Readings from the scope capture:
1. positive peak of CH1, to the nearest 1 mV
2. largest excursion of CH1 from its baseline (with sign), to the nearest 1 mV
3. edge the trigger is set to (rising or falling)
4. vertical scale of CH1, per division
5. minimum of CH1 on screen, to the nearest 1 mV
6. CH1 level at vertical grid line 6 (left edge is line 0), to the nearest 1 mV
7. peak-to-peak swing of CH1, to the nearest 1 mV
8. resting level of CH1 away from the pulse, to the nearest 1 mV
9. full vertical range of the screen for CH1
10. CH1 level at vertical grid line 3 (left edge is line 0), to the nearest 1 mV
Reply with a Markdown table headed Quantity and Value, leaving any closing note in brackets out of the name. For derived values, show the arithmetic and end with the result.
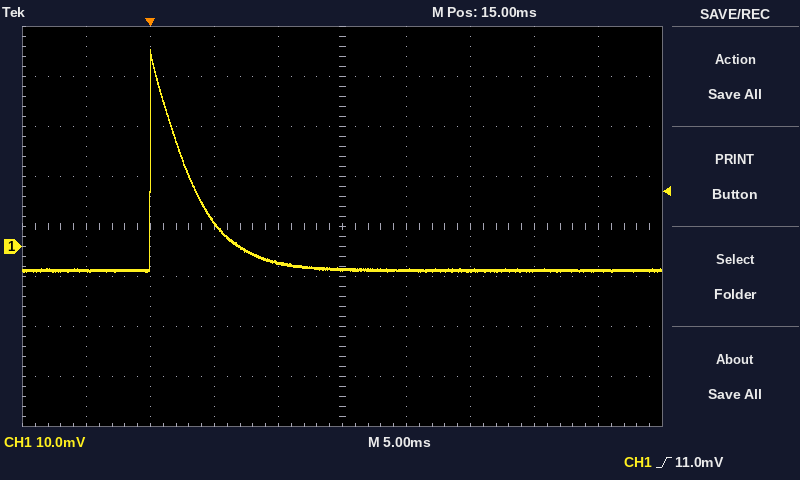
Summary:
| Quantity | Value |
|---|---|
| positive peak of CH1, to the nearest 1 mV | 39 mV |
| largest excursion of CH1 from its baseline (with sign), to the nearest 1 mV | 39 mV − (-5 mV) = +44 mV |
| edge the trigger is set to | rising |
| vertical scale of CH1, per division | 10 mV |
| minimum of CH1 on screen, to the nearest 1 mV | -5 mV |
| CH1 level at vertical grid line 6 (left edge is line 0), to the nearest 1 mV | -5 mV |
| peak-to-peak swing of CH1, to the nearest 1 mV | 39 mV − (-5 mV) = 44 mV |
| resting level of CH1 away from the pulse, to the nearest 1 mV | -5 mV |
| full vertical range of the screen for CH1 | 80 mV |
| CH1 level at vertical grid line 3 (left edge is line 0), to the nearest 1 mV | 5 mV |
